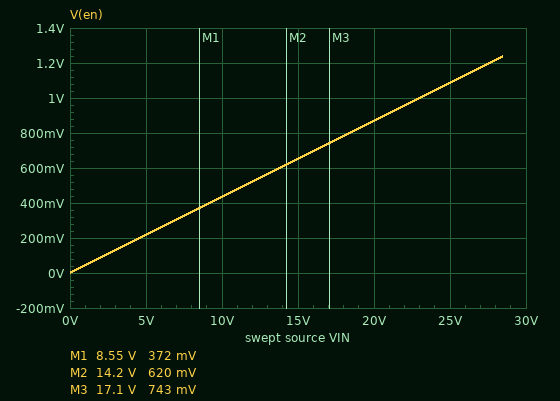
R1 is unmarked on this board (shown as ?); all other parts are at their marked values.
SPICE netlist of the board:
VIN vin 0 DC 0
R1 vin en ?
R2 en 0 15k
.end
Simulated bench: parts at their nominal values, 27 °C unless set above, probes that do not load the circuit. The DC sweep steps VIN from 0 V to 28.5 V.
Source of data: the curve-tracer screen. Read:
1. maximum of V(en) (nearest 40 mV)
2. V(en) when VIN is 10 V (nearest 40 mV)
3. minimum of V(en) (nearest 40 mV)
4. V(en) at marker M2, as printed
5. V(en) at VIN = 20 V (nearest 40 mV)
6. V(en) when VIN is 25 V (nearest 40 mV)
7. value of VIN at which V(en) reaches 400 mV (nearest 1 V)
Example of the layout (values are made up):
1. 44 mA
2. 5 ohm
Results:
1. 1.24 V
2. 440 mV
3. 0 V
4. 620 mV
5. 880 mV
6. 1.08 V
7. 9 V
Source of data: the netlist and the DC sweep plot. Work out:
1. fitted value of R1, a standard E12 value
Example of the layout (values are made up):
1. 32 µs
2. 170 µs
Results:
1. 330 kΩ
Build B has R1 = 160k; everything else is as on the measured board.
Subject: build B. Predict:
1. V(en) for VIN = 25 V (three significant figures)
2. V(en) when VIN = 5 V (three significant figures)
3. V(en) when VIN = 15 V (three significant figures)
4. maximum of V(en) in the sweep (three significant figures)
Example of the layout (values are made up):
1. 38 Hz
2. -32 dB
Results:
1. 2.14 V
2. 429 mV
3. 1.29 V
4. 2.44 V
